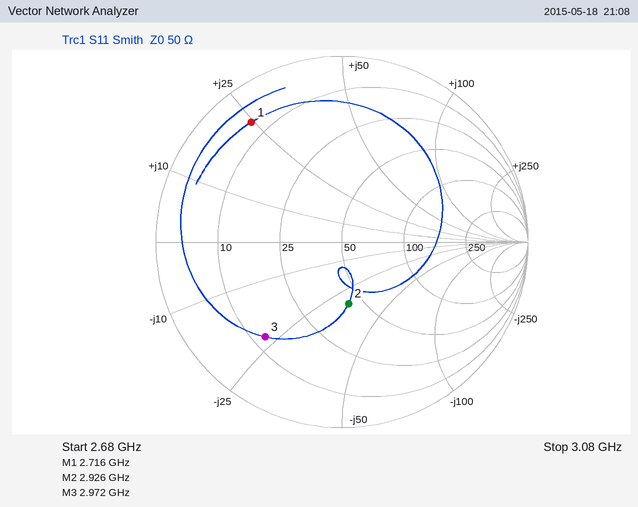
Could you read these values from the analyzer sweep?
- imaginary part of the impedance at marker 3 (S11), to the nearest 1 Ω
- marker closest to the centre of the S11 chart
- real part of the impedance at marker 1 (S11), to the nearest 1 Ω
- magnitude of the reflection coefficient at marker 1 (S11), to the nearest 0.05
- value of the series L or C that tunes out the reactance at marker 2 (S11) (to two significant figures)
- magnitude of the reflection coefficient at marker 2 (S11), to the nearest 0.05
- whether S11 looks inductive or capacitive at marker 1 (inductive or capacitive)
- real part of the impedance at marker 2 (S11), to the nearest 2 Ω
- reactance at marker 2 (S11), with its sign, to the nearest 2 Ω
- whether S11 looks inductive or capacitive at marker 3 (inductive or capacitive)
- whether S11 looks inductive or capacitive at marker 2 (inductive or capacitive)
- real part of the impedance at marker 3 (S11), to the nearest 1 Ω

-23 Ω
marker 2
7 Ω
0.80
1.7 nH
0.35
inductive
42 Ω
-32 Ω
capacitive
capacitive
13 Ω
